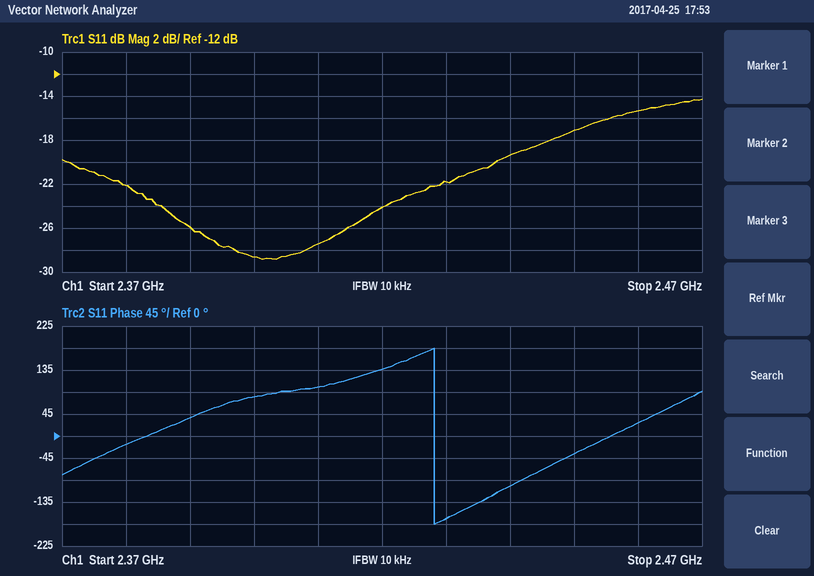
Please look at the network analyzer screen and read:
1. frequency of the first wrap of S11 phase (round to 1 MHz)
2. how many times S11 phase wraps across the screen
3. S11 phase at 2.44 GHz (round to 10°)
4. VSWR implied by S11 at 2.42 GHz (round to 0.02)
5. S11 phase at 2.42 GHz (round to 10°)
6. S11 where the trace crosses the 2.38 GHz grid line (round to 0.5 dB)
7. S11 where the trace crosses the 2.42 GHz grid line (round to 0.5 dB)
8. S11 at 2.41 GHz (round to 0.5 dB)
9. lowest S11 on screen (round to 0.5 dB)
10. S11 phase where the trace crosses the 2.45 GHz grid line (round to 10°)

2.428 GHz
1
-100°
1.14
140°
-22.0 dB
-24.0 dB
-27.5 dB
-29.0 dB
-40°
